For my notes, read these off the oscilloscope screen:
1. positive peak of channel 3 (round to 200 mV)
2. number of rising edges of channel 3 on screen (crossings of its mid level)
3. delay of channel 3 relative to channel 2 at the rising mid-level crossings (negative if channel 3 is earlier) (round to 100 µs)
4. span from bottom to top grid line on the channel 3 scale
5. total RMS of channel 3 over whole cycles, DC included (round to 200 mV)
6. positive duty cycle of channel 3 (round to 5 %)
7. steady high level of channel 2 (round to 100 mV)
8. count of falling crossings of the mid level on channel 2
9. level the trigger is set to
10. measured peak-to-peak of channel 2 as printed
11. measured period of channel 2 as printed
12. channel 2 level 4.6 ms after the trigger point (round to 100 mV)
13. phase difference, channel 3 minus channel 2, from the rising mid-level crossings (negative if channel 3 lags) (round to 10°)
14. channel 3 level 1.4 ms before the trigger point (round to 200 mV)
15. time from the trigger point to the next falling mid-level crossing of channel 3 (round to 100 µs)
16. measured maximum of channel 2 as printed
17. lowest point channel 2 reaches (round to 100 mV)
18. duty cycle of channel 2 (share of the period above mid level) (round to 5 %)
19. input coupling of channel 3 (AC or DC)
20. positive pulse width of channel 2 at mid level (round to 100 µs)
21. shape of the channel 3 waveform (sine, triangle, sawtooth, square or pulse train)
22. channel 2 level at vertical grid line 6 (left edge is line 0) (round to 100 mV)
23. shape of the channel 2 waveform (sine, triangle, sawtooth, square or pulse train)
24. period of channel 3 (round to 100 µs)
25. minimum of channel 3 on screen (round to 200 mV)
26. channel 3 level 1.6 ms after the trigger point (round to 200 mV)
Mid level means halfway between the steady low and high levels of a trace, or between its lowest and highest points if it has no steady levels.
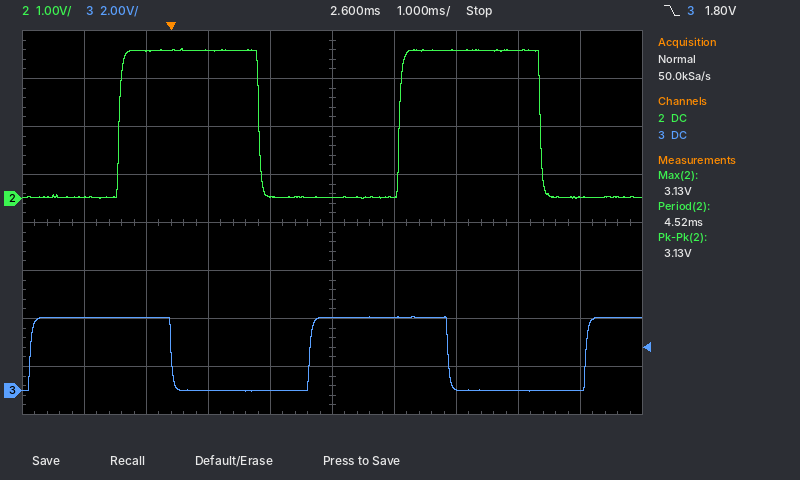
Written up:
3.0 V
3
-1.5 ms
16 V
2.2 V
50 %
3.1 V
2
1.80 V
3.13 V
4.52 ms
3.1 V
+120°
3.0 V
4.5 ms
3.13 V
0.0 V
50 %
DC
2.3 ms
square
100 mV
square
4.5 ms
0.0 V
0.0 V
